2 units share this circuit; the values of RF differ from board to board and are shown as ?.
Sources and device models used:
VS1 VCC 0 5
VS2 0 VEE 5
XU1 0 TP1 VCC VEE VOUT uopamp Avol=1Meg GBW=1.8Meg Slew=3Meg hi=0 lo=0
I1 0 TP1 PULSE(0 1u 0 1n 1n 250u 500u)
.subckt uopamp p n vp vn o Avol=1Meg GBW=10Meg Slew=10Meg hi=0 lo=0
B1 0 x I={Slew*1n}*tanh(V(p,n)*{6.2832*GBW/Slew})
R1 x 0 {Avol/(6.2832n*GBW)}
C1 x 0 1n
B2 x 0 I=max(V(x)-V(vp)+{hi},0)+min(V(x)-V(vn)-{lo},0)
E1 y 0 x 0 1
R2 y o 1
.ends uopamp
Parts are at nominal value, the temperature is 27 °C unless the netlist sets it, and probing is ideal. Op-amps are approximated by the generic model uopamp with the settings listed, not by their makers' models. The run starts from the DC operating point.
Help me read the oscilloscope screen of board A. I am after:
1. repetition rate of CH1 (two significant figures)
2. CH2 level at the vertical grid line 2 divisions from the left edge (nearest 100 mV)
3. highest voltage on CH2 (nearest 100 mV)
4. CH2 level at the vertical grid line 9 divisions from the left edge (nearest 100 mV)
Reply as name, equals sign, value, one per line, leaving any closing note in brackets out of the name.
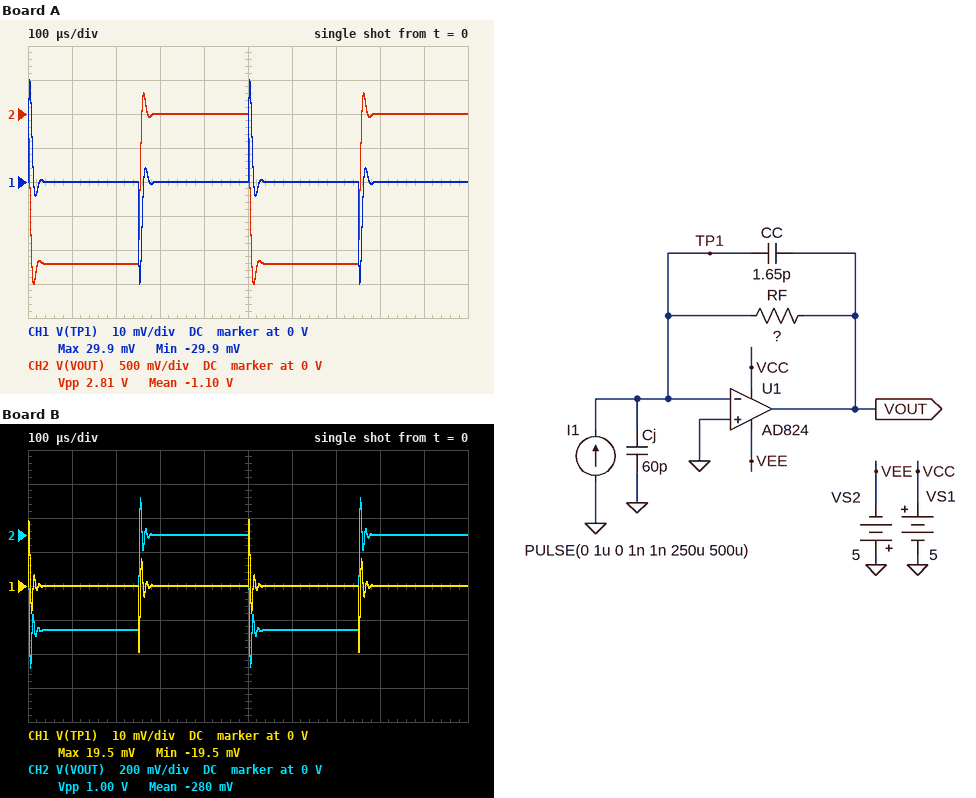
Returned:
repetition rate of CH1 = 2.0 kHz
CH2 level at the vertical grid line 2 divisions from the left edge = -2.2 V
highest voltage on CH2 = 300 mV
CH2 level at the vertical grid line 9 divisions from the left edge = 0 V
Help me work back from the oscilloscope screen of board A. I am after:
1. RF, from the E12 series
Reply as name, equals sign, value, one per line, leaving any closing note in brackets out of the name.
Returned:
RF, from the E12 series = 2.2 MΩ
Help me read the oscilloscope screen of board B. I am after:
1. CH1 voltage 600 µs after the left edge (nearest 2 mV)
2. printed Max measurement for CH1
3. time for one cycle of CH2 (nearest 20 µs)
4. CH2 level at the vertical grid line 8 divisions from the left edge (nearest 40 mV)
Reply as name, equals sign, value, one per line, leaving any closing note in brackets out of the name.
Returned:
CH1 voltage 600 µs after the left edge = 0 V
printed Max measurement for CH1 = 19.5 mV
time for one cycle of CH2 = 500 µs
CH2 level at the vertical grid line 8 divisions from the left edge = 0 V
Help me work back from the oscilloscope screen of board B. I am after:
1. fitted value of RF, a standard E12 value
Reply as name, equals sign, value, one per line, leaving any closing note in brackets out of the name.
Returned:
fitted value of RF, a standard E12 value = 560 kΩ
